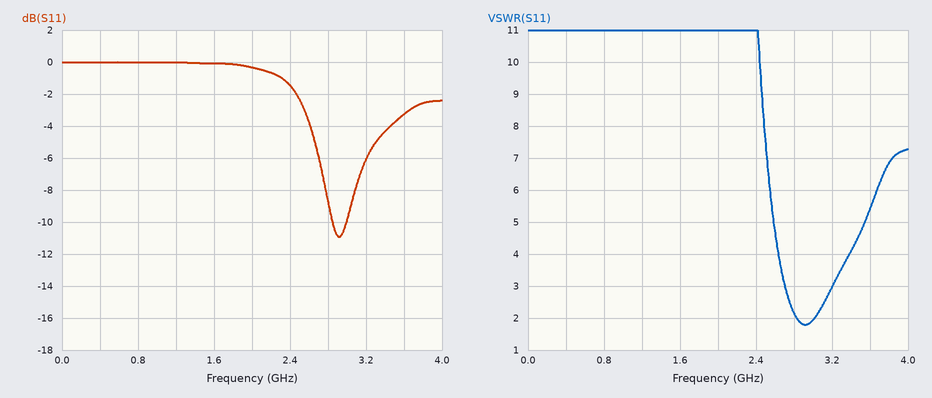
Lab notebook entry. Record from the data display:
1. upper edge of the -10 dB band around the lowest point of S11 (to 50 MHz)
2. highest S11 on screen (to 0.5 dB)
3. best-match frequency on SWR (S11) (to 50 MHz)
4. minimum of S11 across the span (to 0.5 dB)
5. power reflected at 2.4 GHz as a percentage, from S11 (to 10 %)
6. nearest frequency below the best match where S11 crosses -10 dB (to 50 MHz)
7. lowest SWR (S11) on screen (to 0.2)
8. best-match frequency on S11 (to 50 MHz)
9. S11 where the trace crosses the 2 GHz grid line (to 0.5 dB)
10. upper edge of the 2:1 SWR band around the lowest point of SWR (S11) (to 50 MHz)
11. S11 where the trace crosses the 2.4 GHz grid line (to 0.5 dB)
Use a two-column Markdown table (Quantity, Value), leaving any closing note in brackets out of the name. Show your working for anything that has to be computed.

| Quantity | Value |
|---|---|
| upper edge of the -10 dB band around the lowest point of S11 | 3.00 GHz |
| highest S11 on screen | 0.0 dB |
| best-match frequency on SWR (S11) | 2.90 GHz |
| minimum of S11 across the span | -11.0 dB |
| power reflected at 2.4 GHz as a percentage, from S11 | 10^(-1.5/10) ≈ 70.8 %, so 70 % to the nearest 10 % |
| nearest frequency below the best match where S11 crosses -10 dB | 2.85 GHz |
| lowest SWR (S11) on screen | 1.8 |
| best-match frequency on S11 | 2.90 GHz |
| S11 where the trace crosses the 2 GHz grid line | -0.5 dB |
| upper edge of the 2:1 SWR band around the lowest point of SWR (S11) | 3.00 GHz |
| S11 where the trace crosses the 2.4 GHz grid line | -1.5 dB |
